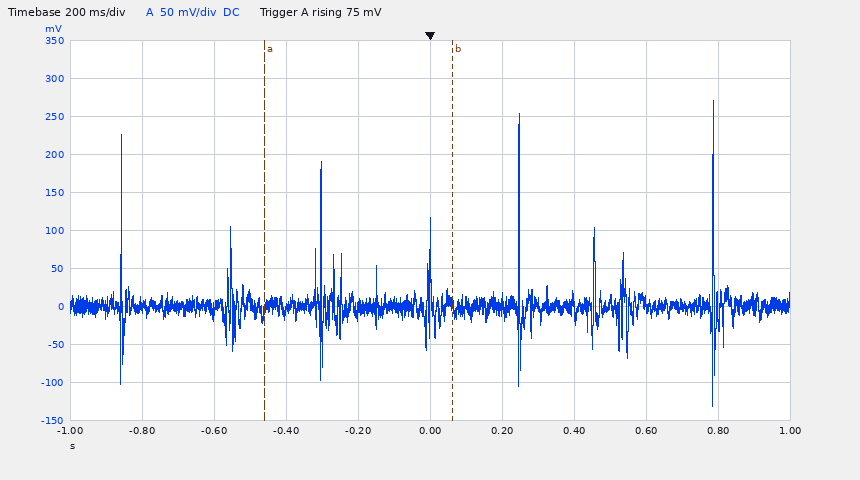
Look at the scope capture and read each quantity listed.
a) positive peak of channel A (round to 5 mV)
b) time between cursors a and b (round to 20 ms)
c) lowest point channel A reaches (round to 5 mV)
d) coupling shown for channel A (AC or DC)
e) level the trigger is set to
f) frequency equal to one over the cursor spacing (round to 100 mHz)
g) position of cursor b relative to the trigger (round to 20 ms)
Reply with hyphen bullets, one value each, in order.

- 270 mV
- 520 ms
- -130 mV
- DC
- 75 mV
- 1.9 Hz
- +60 ms
